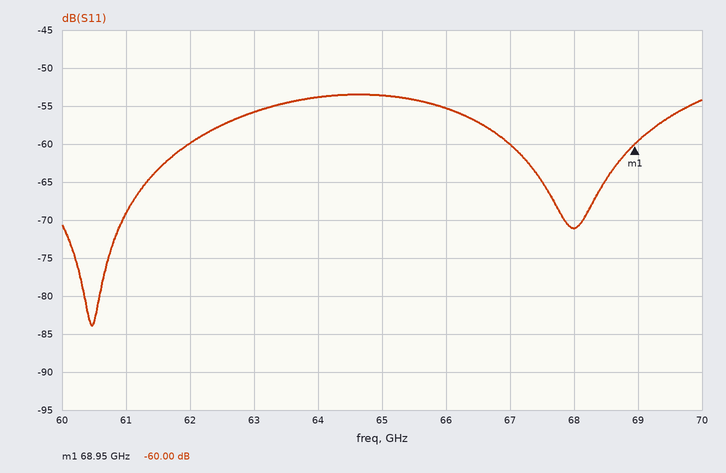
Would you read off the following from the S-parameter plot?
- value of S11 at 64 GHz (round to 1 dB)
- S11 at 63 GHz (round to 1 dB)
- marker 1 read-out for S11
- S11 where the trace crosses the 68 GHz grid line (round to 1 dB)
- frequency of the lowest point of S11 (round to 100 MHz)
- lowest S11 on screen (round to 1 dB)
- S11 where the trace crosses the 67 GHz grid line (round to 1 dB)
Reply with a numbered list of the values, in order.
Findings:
1. -54 dB
2. -56 dB
3. -60.00 dB
4. -71 dB
5. 60.5 GHz
6. -84 dB
7. -60 dB
